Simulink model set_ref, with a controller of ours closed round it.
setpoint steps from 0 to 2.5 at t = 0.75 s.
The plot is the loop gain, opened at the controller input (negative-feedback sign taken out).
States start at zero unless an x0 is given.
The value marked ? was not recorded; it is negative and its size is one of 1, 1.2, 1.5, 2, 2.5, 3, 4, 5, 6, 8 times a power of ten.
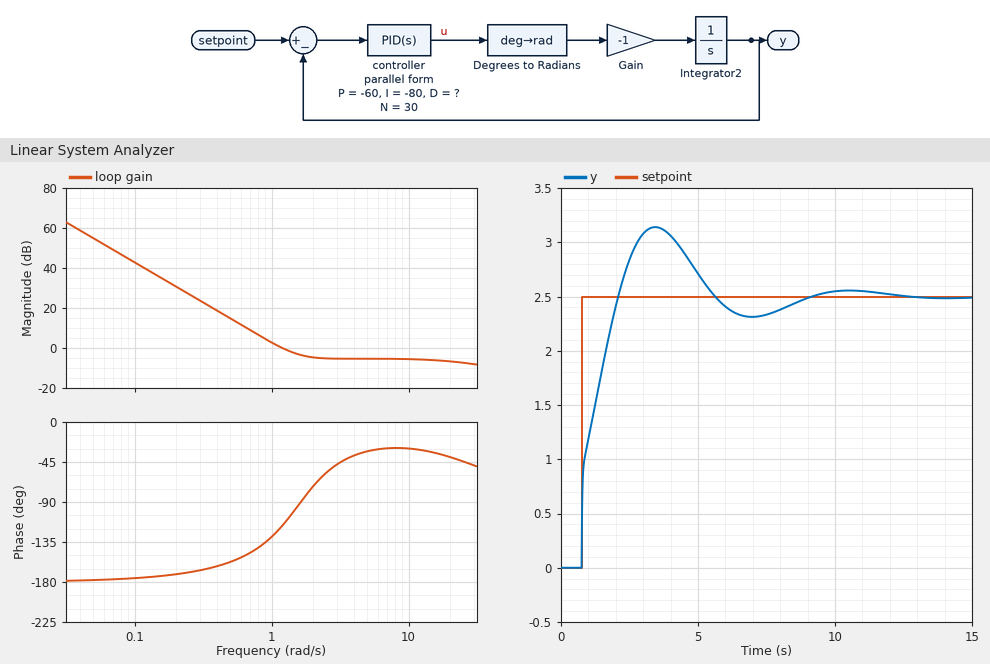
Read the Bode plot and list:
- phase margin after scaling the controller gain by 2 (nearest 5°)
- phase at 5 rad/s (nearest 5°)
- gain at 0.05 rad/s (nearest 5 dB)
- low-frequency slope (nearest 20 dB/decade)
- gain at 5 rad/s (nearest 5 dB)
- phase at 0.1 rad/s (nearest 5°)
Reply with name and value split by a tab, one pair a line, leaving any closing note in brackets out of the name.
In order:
phase margin after scaling the controller gain by 2	145°
phase at 5 rad/s	-35°
gain at 0.05 rad/s	55 dB
low-frequency slope	-40 dB/decade
gain at 5 rad/s	-5 dB
phase at 0.1 rad/s	-175°
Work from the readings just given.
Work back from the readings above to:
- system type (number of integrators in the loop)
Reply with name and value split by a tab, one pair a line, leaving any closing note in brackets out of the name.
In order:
system type	2
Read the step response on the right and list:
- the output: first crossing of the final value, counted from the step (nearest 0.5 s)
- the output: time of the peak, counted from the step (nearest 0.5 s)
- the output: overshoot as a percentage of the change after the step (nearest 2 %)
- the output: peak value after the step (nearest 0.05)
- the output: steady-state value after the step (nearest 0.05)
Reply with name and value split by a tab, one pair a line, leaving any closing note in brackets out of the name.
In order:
the output: first crossing of the final value, counted from the step	1.5 s
the output: time of the peak, counted from the step	2.5 s
the output: overshoot as a percentage of the change after the step	26 %
the output: peak value after the step	3.15
the output: steady-state value after the step	2.50
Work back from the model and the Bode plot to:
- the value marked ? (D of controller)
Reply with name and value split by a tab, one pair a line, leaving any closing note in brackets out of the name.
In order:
the value marked ?	-30
